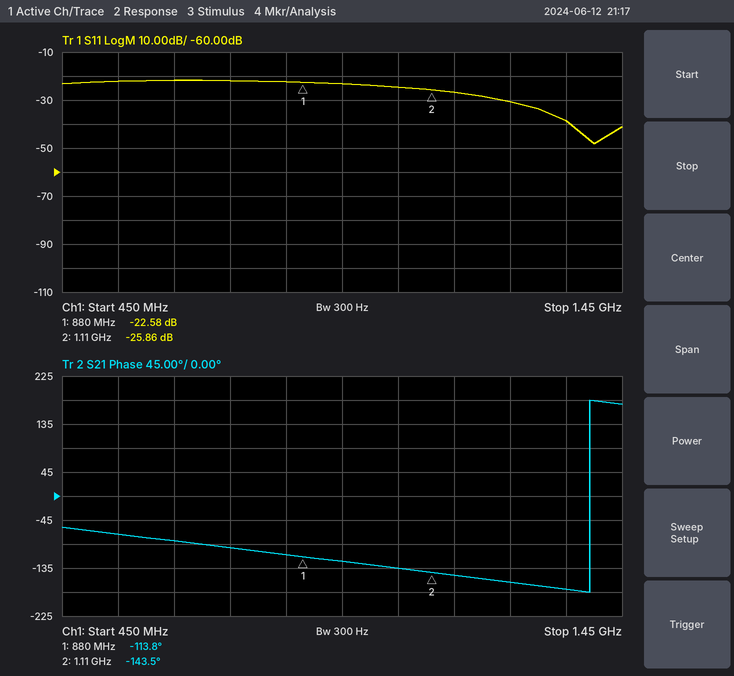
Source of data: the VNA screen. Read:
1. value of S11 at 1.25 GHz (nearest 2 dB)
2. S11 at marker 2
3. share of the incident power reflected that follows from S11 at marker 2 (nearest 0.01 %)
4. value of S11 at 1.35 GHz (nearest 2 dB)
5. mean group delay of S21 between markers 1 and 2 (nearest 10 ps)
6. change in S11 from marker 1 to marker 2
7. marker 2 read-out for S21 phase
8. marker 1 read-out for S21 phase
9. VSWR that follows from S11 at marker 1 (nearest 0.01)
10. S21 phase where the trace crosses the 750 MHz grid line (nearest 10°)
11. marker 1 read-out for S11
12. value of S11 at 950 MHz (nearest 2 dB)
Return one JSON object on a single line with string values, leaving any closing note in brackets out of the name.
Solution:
{"value of S11 at 1.25 GHz": "-30 dB", "S11 at marker 2": "-25.86 dB", "share of the incident power reflected that follows from S11 at marker 2": "0.26 %", "value of S11 at 1.35 GHz": "-38 dB", "mean group delay of S21 between markers 1 and 2": "360 ps", "change in S11 from marker 1 to marker 2": "-3.28 dB", "marker 2 read-out for S21 phase": "-143.5°", "marker 1 read-out for S21 phase": "-113.8°", "VSWR that follows from S11 at marker 1": "1.16", "S21 phase where the trace crosses the 750 MHz grid line": "-100°", "marker 1 read-out for S11": "-22.58 dB", "value of S11 at 950 MHz": "-24 dB"}
